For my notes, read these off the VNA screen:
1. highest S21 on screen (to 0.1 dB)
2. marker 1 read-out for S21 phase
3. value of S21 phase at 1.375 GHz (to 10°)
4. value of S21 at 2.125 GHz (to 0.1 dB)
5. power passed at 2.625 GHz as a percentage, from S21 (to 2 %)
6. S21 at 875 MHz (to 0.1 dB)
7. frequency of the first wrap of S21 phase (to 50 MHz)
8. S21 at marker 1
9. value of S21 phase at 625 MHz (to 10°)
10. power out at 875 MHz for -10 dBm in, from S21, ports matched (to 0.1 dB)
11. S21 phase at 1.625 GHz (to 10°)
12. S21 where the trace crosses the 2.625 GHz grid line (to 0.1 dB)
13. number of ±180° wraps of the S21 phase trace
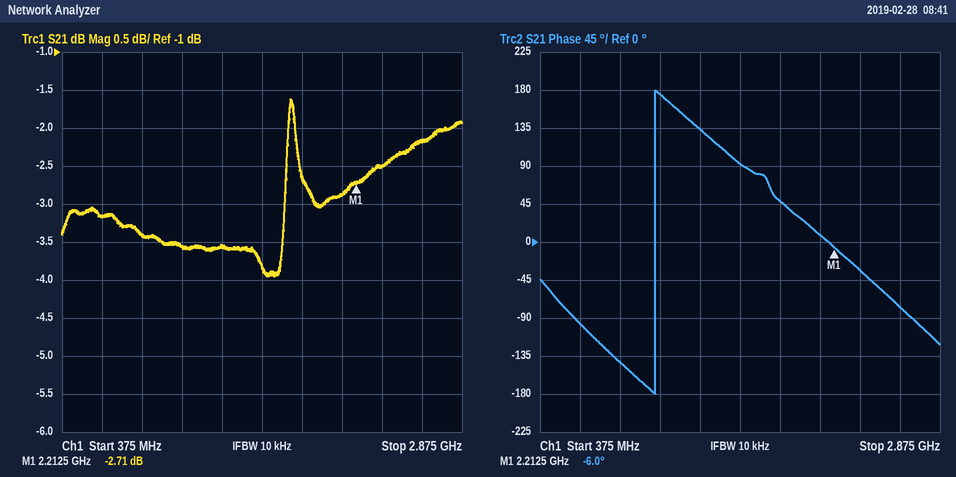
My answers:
-1.6 dB
-6.0°
130°
-2.9 dB
60 %
-3.4 dB
1.10 GHz
-2.71 dB
-100°
-13.4 dBm
90°
-2.2 dB
1
